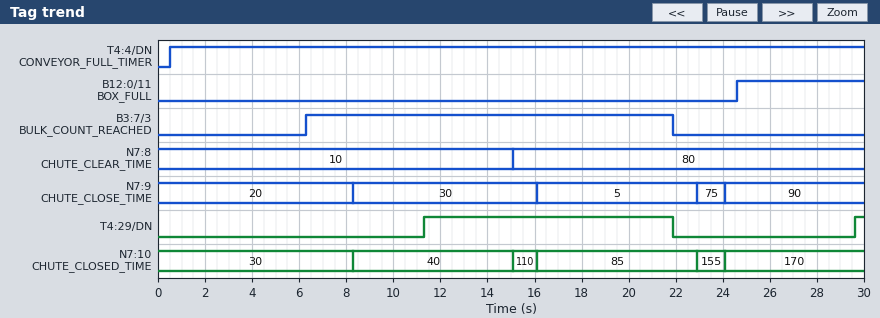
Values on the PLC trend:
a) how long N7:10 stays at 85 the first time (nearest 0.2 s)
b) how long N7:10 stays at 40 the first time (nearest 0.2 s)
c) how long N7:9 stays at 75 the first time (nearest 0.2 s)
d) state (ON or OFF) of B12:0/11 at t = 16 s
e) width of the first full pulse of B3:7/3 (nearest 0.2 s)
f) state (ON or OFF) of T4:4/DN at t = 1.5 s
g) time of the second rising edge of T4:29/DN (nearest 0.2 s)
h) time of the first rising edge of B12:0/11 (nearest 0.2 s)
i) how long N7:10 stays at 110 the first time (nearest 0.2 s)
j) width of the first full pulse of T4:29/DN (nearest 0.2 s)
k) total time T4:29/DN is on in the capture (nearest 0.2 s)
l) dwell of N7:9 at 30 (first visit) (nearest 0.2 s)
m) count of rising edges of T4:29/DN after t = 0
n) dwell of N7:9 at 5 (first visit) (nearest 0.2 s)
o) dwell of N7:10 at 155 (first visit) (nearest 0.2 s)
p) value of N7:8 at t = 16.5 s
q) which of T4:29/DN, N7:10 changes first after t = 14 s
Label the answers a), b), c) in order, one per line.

a) 6.8 s
b) 6.8 s
c) 1.2 s
d) OFF
e) 15.6 s
f) ON
g) 29.6 s
h) 24.6 s
i) 1.0 s
j) 10.6 s
k) 11.0 s
l) 7.8 s
m) 2
n) 6.8 s
o) 1.2 s
p) 80
q) N7:10
